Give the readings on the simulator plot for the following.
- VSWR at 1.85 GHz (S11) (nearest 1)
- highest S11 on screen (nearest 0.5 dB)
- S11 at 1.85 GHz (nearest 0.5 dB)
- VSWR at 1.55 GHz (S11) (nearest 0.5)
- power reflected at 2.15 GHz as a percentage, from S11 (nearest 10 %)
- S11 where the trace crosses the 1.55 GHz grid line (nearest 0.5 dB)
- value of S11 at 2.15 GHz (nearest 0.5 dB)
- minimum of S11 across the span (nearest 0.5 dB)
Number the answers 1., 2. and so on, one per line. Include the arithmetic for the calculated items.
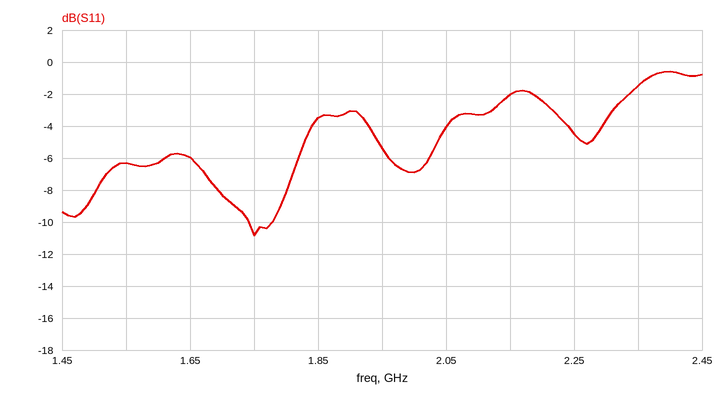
1. |Γ| = 10^(-3.5/20) = 0.6683; VSWR = (1 + 0.6683)/(1 − 0.6683) ≈ 5
2. -0.5 dB
3. -3.5 dB
4. |Γ| = 10^(-6.5/20) = 0.4732; VSWR = (1 + 0.4732)/(1 − 0.4732) ≈ 2.80, so 3.0 to the nearest 0.5
5. 10^(-2/10) ≈ 63.1 %, so 60 % to the nearest 10 %
6. -6.5 dB
7. -2.0 dB
8. -11.0 dB
